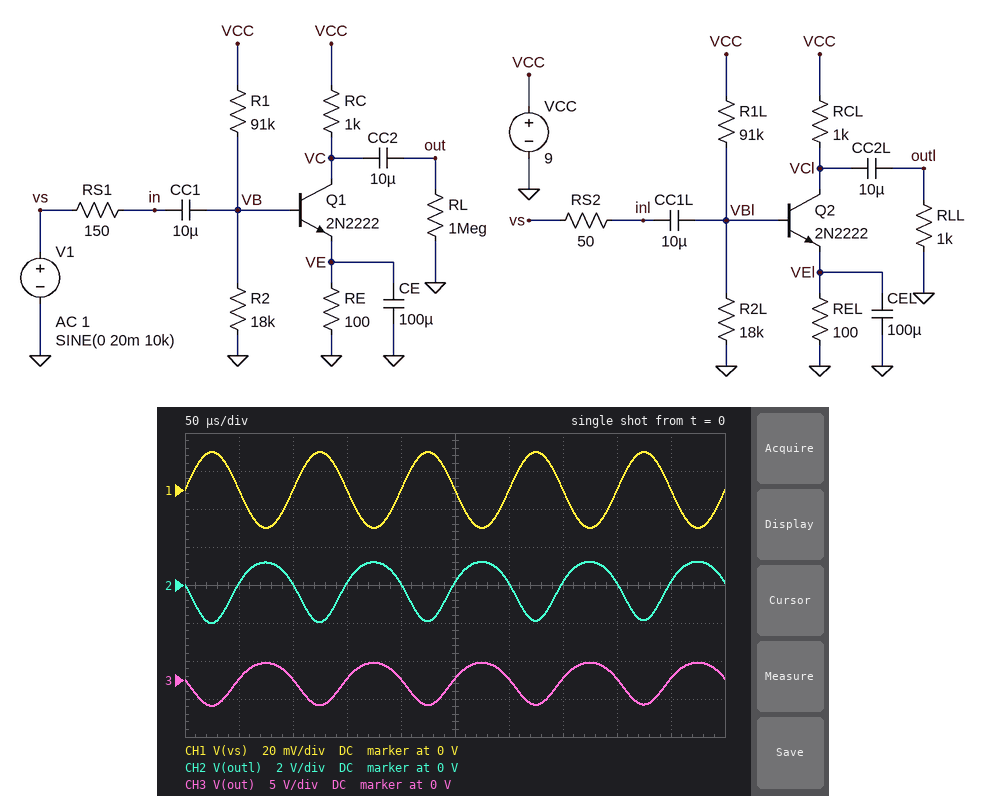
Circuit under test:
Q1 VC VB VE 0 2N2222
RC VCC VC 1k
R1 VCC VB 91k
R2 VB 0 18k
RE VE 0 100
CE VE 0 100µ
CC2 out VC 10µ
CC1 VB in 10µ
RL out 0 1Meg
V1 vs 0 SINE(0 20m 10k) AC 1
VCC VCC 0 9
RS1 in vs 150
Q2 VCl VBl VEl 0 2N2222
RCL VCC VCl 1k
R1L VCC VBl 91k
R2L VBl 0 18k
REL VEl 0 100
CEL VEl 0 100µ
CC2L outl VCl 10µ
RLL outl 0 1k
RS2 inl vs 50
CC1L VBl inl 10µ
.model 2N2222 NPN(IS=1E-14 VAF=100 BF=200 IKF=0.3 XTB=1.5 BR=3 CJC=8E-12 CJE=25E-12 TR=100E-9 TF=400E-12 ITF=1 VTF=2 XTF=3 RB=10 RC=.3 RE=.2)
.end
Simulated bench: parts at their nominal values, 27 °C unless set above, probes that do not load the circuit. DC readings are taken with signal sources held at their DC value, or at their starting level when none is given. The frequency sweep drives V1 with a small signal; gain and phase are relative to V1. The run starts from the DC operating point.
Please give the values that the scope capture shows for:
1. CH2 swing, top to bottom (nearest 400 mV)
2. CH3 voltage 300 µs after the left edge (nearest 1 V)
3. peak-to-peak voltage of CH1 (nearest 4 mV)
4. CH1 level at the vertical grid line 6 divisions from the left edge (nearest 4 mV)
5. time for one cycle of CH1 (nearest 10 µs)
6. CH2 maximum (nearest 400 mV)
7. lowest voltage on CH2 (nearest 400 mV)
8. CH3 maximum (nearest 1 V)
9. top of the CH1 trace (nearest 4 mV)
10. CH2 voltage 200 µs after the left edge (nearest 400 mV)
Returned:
3.2 V
0 V
40 mV
0 V
100 µs
1.2 V
-2.0 V
2 V
20 mV
0 V
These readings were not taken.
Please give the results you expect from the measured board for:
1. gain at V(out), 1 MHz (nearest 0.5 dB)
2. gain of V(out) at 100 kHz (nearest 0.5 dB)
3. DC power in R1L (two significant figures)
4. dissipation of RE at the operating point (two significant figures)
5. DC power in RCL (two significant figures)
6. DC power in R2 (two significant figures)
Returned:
41.0 dB
43.0 dB
680 µW
2.1 mW
21 mW
74 µW
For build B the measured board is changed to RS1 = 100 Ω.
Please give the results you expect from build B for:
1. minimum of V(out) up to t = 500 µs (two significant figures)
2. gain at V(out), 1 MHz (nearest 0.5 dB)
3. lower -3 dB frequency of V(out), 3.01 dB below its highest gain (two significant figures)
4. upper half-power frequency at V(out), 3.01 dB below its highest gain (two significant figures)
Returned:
-3.6 V
42.0 dB
260 Hz
1.8 MHz
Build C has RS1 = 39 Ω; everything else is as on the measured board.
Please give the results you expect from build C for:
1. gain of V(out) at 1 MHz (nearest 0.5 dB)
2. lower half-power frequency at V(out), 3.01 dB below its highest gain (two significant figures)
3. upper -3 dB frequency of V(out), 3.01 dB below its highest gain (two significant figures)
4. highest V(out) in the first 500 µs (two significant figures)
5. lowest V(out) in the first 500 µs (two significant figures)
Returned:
43.5 dB
270 Hz
3.7 MHz
2.4 V
-3.8 V
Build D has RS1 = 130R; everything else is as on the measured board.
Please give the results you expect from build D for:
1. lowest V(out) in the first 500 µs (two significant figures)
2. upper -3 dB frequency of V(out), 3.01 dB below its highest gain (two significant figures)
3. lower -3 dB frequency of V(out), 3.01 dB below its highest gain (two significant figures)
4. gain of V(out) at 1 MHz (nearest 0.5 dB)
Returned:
-3.5 V
1.5 MHz
260 Hz
41.5 dB
